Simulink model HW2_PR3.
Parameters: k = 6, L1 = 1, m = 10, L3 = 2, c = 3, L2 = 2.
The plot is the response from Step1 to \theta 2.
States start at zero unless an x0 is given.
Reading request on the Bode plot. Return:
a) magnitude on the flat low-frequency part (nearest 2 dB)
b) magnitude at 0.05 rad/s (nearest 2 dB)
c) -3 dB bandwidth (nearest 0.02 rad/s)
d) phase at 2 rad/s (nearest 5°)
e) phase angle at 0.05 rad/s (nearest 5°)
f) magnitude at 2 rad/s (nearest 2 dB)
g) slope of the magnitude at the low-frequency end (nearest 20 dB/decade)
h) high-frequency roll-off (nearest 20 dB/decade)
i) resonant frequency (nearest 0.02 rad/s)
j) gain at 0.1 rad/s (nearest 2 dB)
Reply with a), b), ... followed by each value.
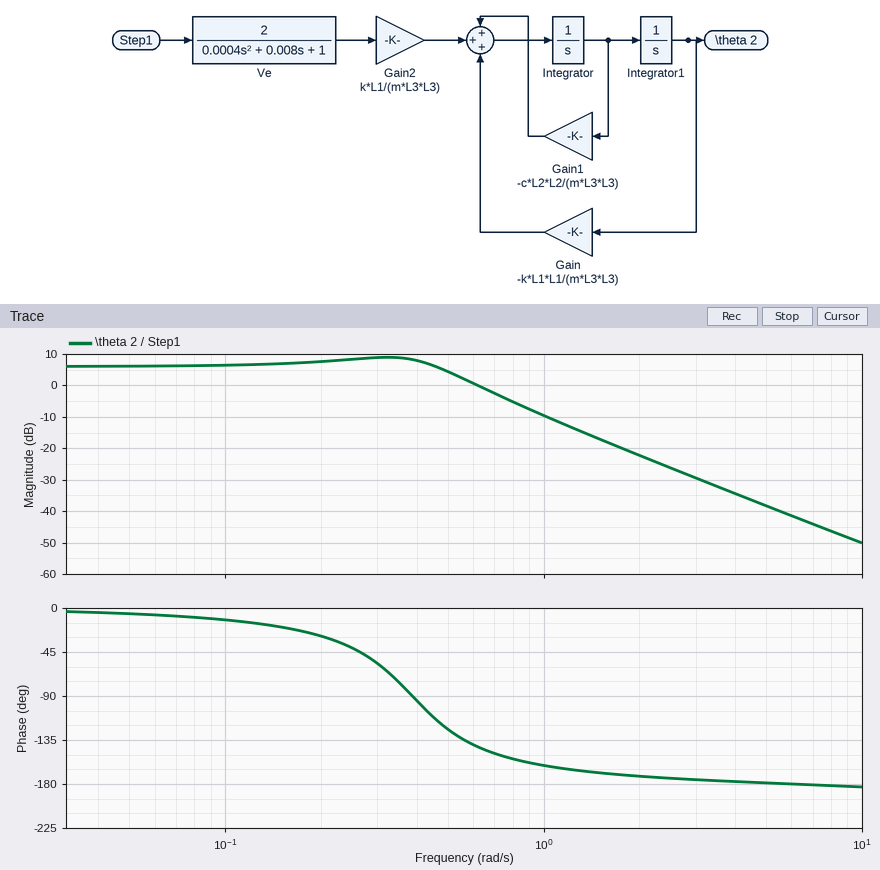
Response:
a) 6 dB
b) 6 dB
c) 0.54 rad/s
d) -170°
e) -5°
f) -22 dB
g) 0 dB/decade
h) -40 dB/decade
i) 0.32 rad/s
j) 6 dB
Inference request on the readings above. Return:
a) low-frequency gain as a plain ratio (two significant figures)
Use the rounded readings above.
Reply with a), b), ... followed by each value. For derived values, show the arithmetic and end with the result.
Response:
a) 10^(6 / 20) = 2.0
